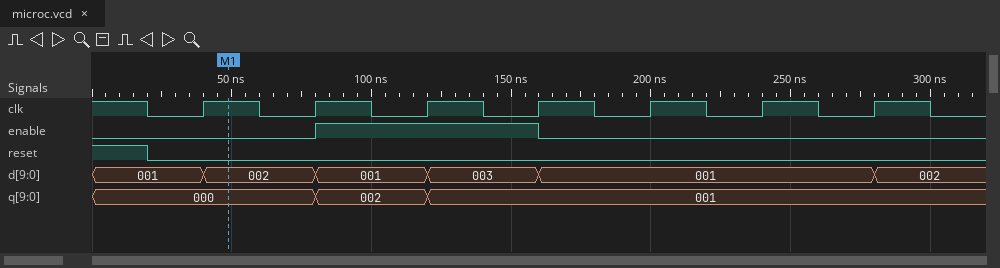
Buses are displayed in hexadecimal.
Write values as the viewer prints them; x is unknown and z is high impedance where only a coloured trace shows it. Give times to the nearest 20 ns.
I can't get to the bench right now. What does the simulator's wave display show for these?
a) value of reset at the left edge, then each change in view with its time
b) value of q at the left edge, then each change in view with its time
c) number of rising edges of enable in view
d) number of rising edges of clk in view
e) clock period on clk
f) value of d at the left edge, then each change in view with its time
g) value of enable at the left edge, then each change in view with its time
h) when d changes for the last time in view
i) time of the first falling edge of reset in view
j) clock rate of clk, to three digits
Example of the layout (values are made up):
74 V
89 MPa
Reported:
1, 0 at 20 ns
000, 002 at 80 ns, 001 at 120 ns
1
7
40 ns
001, 002 at 40 ns, 001 at 80 ns, 003 at 120 ns, 001 at 160 ns, 002 at 280 ns
0, 1 at 80 ns, 0 at 160 ns
280 ns
20 ns
25.0 MHz
